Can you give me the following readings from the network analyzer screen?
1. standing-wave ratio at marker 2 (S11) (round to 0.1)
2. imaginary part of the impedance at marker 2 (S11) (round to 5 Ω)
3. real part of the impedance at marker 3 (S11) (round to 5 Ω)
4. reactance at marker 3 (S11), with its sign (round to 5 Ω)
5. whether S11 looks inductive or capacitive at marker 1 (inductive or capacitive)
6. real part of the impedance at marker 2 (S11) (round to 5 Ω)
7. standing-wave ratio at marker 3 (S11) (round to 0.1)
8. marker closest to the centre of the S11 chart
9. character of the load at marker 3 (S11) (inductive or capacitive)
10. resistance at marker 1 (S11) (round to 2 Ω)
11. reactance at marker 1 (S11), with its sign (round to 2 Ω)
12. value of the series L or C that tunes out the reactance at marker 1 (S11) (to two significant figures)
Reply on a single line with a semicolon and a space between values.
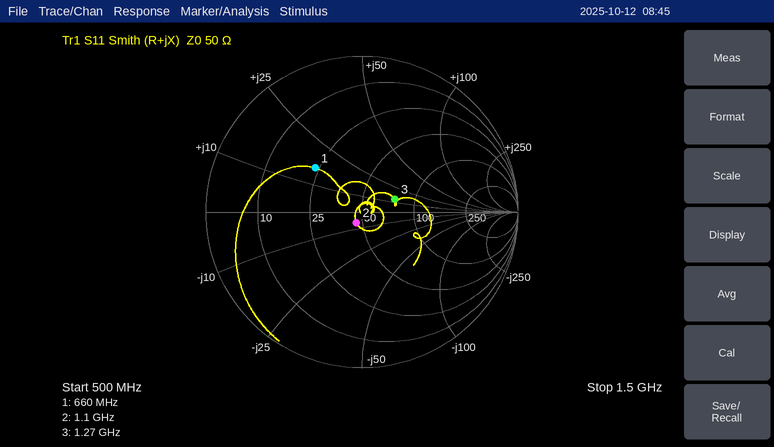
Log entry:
1.2; -5 Ω; 75 Ω; +15 Ω; inductive; 45 Ω; 1.6; marker 2; inductive; 24 Ω; +16 Ω; 15 pF
